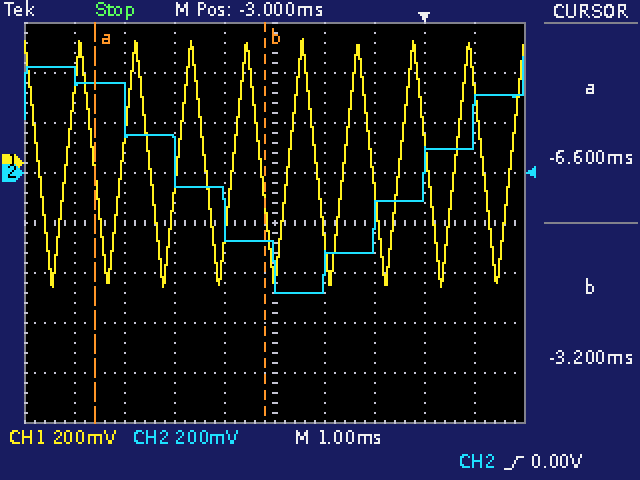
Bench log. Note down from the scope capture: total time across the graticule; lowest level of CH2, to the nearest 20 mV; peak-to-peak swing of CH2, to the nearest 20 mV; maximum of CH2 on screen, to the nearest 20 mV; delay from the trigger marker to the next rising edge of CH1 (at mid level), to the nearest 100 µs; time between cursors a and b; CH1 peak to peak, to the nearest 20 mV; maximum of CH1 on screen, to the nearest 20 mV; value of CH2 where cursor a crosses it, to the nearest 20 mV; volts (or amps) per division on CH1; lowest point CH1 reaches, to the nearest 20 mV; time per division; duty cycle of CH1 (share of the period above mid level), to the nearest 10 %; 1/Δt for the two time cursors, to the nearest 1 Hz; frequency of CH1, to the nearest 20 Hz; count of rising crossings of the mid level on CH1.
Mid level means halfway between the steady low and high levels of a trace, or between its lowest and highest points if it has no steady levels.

10 ms
-480 mV
940 mV
460 mV
600 µs
3.4 ms
1.00 V
500 mV
360 mV
200 mV
-500 mV
1 ms
50 %
294 Hz
900 Hz
9
